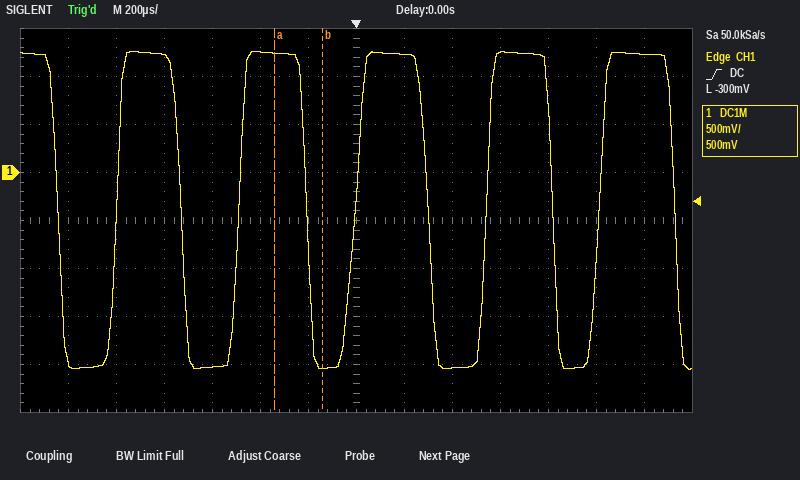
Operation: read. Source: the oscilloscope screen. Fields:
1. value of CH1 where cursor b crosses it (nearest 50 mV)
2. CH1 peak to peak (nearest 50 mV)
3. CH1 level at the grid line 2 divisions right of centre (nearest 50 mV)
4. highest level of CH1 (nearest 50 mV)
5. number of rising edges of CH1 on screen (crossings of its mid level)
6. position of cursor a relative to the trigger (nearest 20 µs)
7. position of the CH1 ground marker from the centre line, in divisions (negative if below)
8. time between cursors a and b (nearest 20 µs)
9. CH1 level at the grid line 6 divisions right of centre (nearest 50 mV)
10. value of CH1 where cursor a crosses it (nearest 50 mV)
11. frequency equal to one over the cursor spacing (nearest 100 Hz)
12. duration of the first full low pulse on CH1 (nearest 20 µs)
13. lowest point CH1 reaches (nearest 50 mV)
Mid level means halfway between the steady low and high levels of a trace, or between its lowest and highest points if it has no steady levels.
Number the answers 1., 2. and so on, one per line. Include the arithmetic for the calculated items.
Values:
1. -2.05 V
2. 1.25 V − (-2.05 V) = 3.30 V
3. -2.05 V
4. 1.25 V
5. 5
6. -340 µs
7. +1.0 div
8. 200 µs
9. 1.25 V
10. 1.25 V
11. 1 / 200 µs ≈ 5.0 kHz
12. 240 µs
13. -2.05 V
